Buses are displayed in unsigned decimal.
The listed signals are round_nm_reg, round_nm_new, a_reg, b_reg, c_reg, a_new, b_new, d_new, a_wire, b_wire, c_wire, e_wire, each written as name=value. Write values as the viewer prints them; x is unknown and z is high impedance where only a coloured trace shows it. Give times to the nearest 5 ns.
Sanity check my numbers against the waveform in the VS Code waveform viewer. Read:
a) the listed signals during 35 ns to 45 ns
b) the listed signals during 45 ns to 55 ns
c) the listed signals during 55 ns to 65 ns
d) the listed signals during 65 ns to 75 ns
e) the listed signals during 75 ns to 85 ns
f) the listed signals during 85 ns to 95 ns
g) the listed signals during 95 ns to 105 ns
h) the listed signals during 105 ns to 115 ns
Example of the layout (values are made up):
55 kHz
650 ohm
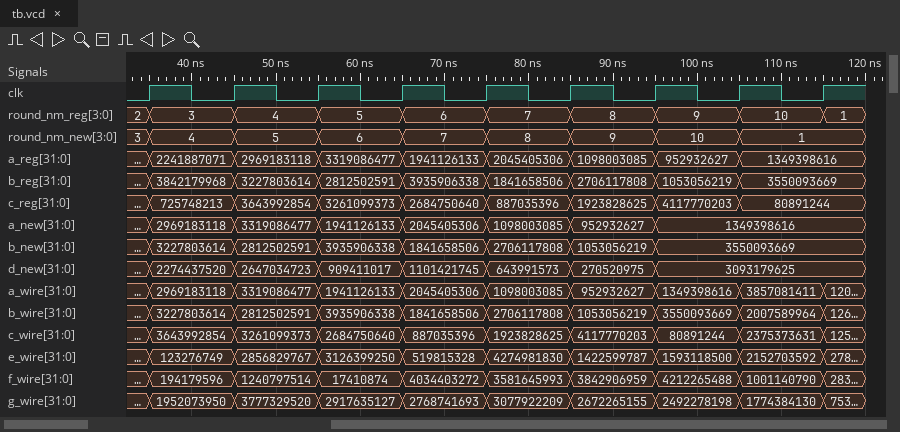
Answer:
round_nm_reg=3, round_nm_new=4, a_reg=2241887071, b_reg=3842179968, c_reg=725748213, a_new=2969183118, b_new=3227803614, d_new=2274437520, a_wire=2969183118, b_wire=3227803614, c_wire=3643992854, e_wire=123276749
round_nm_reg=4, round_nm_new=5, a_reg=2969183118, b_reg=3227803614, c_reg=3643992854, a_new=3319086477, b_new=2812502591, d_new=2647034723, a_wire=3319086477, b_wire=2812502591, c_wire=3261099373, e_wire=2856829767
round_nm_reg=5, round_nm_new=6, a_reg=3319086477, b_reg=2812502591, c_reg=3261099373, a_new=1941126133, b_new=3935906338, d_new=909411017, a_wire=1941126133, b_wire=3935906338, c_wire=2684750640, e_wire=3126399250
round_nm_reg=6, round_nm_new=7, a_reg=1941126133, b_reg=3935906338, c_reg=2684750640, a_new=2045405306, b_new=1841658506, d_new=1101421745, a_wire=2045405306, b_wire=1841658506, c_wire=887035396, e_wire=519815328
round_nm_reg=7, round_nm_new=8, a_reg=2045405306, b_reg=1841658506, c_reg=887035396, a_new=1098003085, b_new=2706117808, d_new=643991573, a_wire=1098003085, b_wire=2706117808, c_wire=1923828625, e_wire=4274981830
round_nm_reg=8, round_nm_new=9, a_reg=1098003085, b_reg=2706117808, c_reg=1923828625, a_new=952932627, b_new=1053056219, d_new=270520975, a_wire=952932627, b_wire=1053056219, c_wire=4117770203, e_wire=1422599787
round_nm_reg=9, round_nm_new=10, a_reg=952932627, b_reg=1053056219, c_reg=4117770203, a_new=1349398616, b_new=3550093669, d_new=3093179625, a_wire=1349398616, b_wire=3550093669, c_wire=80891244, e_wire=1593118500
round_nm_reg=10, round_nm_new=1, a_reg=1349398616, b_reg=3550093669, c_reg=80891244, a_new=1349398616, b_new=3550093669, d_new=3093179625, a_wire=3857081411, b_wire=2007589964, c_wire=2375373631, e_wire=2152703592
